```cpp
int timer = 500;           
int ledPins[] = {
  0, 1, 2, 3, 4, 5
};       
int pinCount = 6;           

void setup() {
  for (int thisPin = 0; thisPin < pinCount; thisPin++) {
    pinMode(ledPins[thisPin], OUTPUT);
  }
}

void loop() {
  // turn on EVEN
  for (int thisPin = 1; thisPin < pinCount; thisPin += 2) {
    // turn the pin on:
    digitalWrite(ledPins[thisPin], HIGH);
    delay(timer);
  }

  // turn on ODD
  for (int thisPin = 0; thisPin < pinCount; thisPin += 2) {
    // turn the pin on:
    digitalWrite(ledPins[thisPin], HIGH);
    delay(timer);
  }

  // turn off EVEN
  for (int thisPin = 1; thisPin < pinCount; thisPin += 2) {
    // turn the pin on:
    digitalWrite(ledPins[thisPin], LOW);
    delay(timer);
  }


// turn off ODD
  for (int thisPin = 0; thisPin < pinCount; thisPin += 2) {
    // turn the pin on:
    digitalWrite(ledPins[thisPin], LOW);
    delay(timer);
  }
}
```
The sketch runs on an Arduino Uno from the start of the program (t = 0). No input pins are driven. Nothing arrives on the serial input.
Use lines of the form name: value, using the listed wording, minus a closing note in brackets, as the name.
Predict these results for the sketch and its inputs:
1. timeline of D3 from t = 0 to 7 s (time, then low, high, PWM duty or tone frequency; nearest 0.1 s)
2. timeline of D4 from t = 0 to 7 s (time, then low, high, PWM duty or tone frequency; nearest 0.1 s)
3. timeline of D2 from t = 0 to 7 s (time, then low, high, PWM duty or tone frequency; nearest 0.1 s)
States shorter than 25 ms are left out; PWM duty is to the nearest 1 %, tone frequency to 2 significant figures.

timeline of D3 from t = 0 to 7 s: 0 s low; 0.5 s high; 3.5 s low; 6.5 s high
timeline of D4 from t = 0 to 7 s: 0 s low; 2.5 s high; 5.5 s low
timeline of D2 from t = 0 to 7 s: 0 s low; 2 s high; 5 s low
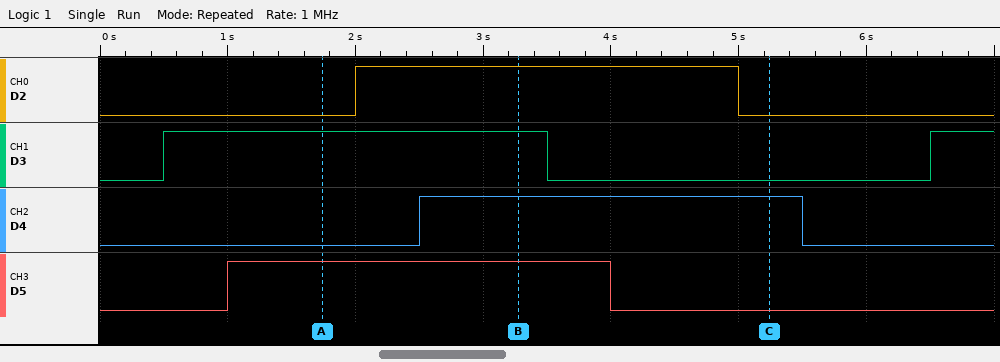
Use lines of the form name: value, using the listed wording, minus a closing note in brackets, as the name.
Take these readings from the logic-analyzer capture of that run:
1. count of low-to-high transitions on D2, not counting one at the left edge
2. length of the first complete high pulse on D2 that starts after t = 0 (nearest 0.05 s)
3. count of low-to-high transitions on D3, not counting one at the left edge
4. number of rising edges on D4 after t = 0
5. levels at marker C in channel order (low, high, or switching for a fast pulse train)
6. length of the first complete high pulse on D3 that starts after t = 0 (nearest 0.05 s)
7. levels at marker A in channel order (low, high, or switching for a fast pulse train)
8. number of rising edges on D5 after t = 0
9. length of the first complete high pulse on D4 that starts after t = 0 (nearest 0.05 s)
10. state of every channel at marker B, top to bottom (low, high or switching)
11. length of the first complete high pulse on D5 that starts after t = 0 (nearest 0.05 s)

count of low-to-high transitions on D2, not counting one at the left edge: 1
length of the first complete high pulse on D2 that starts after t = 0: 3.00 s
count of low-to-high transitions on D3, not counting one at the left edge: 2
number of rising edges on D4 after t = 0: 1
levels at marker C in channel order: D2 low, D3 low, D4 high, D5 low
length of the first complete high pulse on D3 that starts after t = 0: 3.00 s
levels at marker A in channel order: D2 low, D3 high, D4 low, D5 high
number of rising edges on D5 after t = 0: 1
length of the first complete high pulse on D4 that starts after t = 0: 3.00 s
state of every channel at marker B, top to bottom: D2 high, D3 high, D4 high, D5 high
length of the first complete high pulse on D5 that starts after t = 0: 3.00 s
